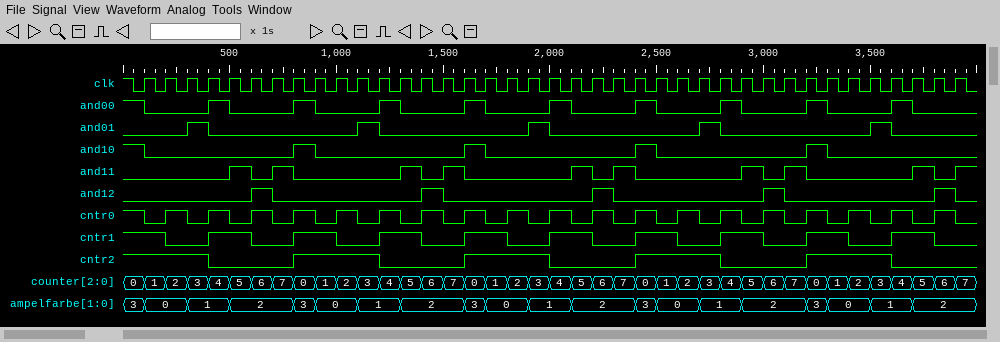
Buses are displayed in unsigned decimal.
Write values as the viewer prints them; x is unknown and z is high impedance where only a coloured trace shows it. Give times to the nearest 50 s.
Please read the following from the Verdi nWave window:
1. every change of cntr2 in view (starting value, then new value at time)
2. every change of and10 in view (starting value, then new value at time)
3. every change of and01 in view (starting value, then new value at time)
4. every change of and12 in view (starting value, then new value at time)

1, 0 at 400 s, 1 at 800 s, 0 at 1200 s, 1 at 1600 s, 0 at 2000 s, 1 at 2400 s, 0 at 2800 s, 1 at 3200 s, 0 at 3600 s
1, 0 at 100 s, 1 at 800 s, 0 at 900 s, 1 at 1600 s, 0 at 1700 s, 1 at 2400 s, 0 at 2500 s, 1 at 3200 s, 0 at 3300 s
0, 1 at 300 s, 0 at 400 s, 1 at 1100 s, 0 at 1200 s, 1 at 1900 s, 0 at 2000 s, 1 at 2700 s, 0 at 2800 s, 1 at 3500 s, 0 at 3600 s
0, 1 at 600 s, 0 at 700 s, 1 at 1400 s, 0 at 1500 s, 1 at 2200 s, 0 at 2300 s, 1 at 3000 s, 0 at 3100 s, 1 at 3800 s, 0 at 3900 s
